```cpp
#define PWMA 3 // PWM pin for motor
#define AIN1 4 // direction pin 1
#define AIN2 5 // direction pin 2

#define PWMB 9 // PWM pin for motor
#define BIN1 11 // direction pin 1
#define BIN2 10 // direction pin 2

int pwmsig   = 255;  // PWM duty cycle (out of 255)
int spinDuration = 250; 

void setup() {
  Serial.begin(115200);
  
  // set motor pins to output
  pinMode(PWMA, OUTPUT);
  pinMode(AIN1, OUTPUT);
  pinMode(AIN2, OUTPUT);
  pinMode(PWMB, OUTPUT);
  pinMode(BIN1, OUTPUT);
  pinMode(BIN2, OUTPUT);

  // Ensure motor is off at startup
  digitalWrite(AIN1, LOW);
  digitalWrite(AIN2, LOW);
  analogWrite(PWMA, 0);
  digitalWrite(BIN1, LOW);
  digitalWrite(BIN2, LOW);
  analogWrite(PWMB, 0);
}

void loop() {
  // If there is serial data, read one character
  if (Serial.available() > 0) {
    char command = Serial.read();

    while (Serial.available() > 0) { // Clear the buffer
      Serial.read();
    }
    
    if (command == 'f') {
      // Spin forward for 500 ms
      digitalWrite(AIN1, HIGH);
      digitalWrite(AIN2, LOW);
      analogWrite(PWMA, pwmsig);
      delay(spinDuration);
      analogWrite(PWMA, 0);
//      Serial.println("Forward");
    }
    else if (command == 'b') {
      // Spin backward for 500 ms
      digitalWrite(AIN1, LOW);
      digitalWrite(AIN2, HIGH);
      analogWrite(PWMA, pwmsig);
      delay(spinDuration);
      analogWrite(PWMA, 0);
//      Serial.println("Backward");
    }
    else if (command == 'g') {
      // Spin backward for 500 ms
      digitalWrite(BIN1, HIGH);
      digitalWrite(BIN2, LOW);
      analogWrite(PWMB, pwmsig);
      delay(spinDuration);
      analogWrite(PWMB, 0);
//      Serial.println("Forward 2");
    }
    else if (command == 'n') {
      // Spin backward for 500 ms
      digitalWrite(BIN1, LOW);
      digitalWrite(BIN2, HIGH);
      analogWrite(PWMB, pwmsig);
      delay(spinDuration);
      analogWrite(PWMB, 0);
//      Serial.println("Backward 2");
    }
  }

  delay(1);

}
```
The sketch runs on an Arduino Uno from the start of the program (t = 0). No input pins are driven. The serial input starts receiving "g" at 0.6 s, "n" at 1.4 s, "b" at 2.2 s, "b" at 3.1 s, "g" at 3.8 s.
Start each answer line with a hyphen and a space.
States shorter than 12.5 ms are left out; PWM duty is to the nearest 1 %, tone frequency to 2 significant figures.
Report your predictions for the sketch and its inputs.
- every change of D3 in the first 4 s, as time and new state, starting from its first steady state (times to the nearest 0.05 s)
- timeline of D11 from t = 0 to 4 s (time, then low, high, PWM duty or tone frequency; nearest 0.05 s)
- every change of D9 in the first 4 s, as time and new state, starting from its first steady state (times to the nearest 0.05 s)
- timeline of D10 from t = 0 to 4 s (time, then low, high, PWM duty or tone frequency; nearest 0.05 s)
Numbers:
- 0 s low; 2.2 s high; 2.45 s low; 3.1 s high; 3.35 s low
- 0 s low; 0.6 s high; 1.4 s low; 3.8 s high
- 0 s low; 0.6 s high; 0.85 s low; 1.4 s high; 1.65 s low; 3.8 s high
- 0 s low; 1.4 s high; 3.8 s low
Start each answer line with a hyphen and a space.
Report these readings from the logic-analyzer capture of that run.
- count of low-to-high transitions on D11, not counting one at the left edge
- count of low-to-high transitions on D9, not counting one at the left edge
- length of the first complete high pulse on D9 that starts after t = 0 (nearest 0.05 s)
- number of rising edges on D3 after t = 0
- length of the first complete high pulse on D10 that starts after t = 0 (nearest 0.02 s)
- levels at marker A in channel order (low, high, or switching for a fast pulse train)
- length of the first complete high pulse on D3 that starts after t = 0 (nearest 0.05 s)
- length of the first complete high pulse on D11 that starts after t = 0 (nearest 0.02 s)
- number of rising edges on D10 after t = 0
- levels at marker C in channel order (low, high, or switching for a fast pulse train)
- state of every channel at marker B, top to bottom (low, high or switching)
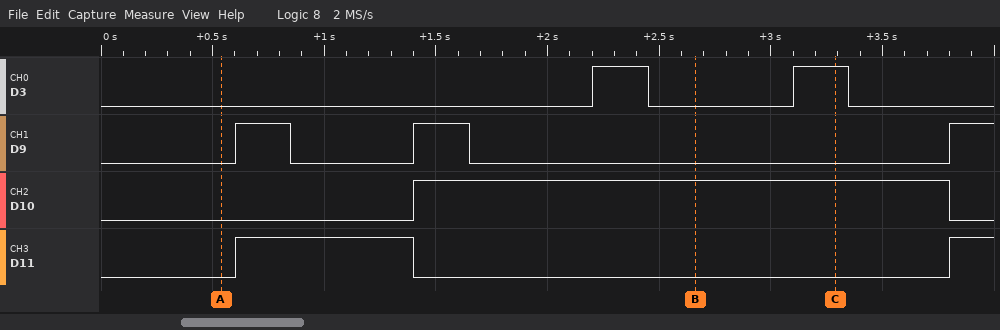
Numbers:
- 2
- 3
- 0.25 s
- 2
- 2.40 s
- D3 low, D9 low, D10 low, D11 low
- 0.25 s
- 0.80 s
- 1
- D3 high, D9 low, D10 high, D11 low
- D3 low, D9 low, D10 high, D11 low
